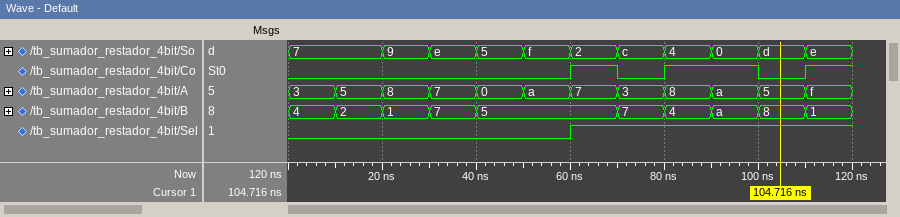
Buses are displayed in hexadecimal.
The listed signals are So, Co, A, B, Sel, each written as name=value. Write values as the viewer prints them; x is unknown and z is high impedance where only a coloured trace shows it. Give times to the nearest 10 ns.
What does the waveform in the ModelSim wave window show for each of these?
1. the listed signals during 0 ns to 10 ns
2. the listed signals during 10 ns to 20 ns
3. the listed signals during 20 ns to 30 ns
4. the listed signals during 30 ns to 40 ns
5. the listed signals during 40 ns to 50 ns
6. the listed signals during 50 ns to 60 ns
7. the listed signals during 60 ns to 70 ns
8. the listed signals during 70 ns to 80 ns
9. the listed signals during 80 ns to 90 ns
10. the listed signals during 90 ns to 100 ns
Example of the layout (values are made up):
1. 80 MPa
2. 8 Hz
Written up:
1. So=7, Co=0, A=3, B=4, Sel=0
2. So=7, Co=0, A=5, B=2, Sel=0
3. So=9, Co=0, A=8, B=1, Sel=0
4. So=e, Co=0, A=7, B=7, Sel=0
5. So=5, Co=0, A=0, B=5, Sel=0
6. So=f, Co=0, A=a, B=5, Sel=0
7. So=2, Co=1, A=7, B=5, Sel=1
8. So=c, Co=0, A=3, B=7, Sel=1
9. So=4, Co=1, A=8, B=4, Sel=1
10. So=0, Co=1, A=a, B=a, Sel=1
